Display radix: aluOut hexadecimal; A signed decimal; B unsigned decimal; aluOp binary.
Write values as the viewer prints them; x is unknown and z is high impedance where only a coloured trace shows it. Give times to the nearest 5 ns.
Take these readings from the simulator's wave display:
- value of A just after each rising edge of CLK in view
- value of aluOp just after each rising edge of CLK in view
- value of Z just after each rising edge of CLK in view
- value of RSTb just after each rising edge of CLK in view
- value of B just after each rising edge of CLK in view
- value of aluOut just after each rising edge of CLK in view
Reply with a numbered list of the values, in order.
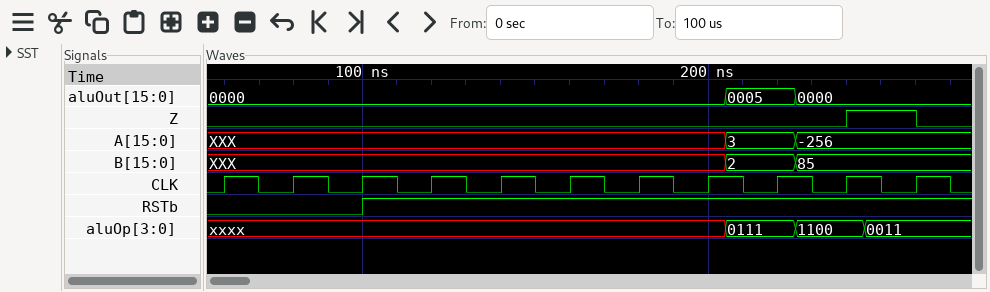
1. XXX, XXX, XXX, XXX, XXX, XXX, XXX, XXX, 3, -256, -256
2. xxxx, xxxx, xxxx, xxxx, xxxx, xxxx, xxxx, xxxx, 0111, 1100, 0011
3. 0 0 0 0 0 0 0 0 0 1 0
4. 0 0 1 1 1 1 1 1 1 1 1
5. XXX, XXX, XXX, XXX, XXX, XXX, XXX, XXX, 2, 85, 85
6. 0000, 0000, 0000, 0000, 0000, 0000, 0000, 0000, 0005, 0000, 0000
